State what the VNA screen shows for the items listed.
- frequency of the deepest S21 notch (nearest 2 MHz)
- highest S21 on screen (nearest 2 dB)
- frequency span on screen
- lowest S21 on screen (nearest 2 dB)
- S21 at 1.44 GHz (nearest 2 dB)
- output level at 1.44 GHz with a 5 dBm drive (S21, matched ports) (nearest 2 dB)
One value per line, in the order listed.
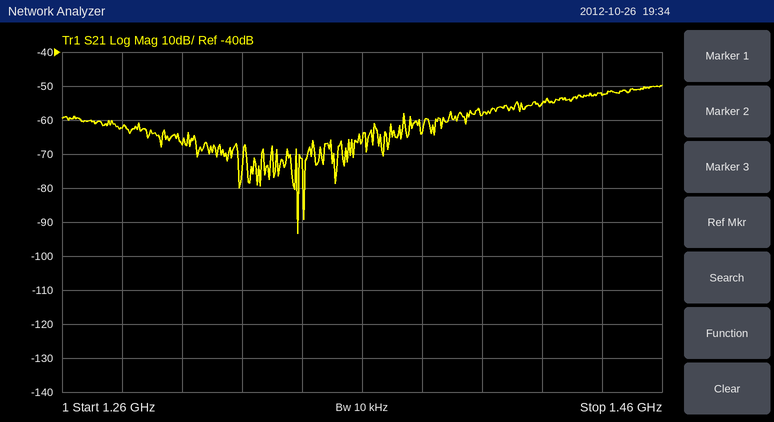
1.338 GHz
-50 dB
200 MHz
-94 dB
-52 dB
-48 dBm
